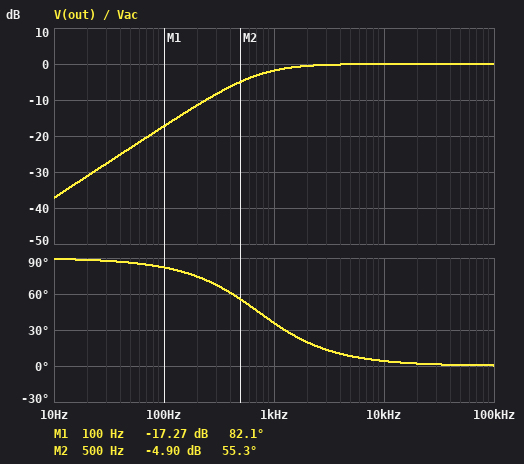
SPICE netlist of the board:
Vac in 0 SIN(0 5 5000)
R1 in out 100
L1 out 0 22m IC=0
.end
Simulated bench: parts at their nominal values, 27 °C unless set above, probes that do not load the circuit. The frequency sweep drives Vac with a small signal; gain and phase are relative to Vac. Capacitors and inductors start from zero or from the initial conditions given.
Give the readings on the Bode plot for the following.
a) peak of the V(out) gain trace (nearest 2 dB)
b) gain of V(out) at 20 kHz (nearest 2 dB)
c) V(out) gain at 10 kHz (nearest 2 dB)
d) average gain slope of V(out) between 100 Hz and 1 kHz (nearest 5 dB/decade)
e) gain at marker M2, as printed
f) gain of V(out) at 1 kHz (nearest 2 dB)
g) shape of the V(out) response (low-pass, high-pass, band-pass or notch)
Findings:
0 dB
0 dB
0 dB
15 dB/decade
-4.90 dB
-2 dB
high-pass
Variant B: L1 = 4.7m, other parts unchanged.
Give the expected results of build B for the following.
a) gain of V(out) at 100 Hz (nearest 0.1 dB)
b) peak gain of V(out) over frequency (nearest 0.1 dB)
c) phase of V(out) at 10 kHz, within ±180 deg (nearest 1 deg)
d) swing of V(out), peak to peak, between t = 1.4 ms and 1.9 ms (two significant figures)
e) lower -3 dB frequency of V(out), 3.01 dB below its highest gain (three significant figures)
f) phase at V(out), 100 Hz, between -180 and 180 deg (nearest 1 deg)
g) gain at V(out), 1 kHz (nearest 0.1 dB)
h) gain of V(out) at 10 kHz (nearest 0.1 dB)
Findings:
-30.6 dB
0 dB
19 deg
8.3 V
3.39 kHz
88 deg
-11.0 dB
-0.5 dB
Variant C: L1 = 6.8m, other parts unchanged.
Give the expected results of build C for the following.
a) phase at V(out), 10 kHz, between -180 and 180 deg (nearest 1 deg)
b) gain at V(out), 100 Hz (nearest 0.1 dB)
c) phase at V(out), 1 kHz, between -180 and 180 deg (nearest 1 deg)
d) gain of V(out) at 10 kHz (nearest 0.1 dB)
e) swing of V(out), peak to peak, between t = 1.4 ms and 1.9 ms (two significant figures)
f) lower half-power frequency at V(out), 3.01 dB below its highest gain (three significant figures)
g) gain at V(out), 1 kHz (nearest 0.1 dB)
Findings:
13 deg
-27.4 dB
67 deg
-0.2 dB
9.1 V
2.34 kHz
-8.1 dB
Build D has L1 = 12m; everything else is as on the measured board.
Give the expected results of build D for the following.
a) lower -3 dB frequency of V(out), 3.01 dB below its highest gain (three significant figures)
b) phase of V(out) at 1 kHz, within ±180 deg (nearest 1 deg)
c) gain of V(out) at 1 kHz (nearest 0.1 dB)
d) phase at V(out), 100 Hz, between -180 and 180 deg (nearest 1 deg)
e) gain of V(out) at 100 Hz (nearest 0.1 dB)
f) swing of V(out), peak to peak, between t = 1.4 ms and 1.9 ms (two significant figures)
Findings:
1.33 kHz
53 deg
-4.4 dB
86 deg
-22.5 dB
9.7 V
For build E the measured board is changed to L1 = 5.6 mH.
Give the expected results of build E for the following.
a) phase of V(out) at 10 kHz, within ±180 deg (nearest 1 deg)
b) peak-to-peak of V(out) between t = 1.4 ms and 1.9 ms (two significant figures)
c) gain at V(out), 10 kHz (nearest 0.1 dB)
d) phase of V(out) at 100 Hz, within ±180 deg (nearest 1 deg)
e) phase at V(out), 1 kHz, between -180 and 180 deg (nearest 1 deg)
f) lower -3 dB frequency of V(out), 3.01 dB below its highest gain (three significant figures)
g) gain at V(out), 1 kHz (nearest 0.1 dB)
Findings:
16 deg
8.7 V
-0.3 dB
88 deg
71 deg
2.84 kHz
-9.6 dB
